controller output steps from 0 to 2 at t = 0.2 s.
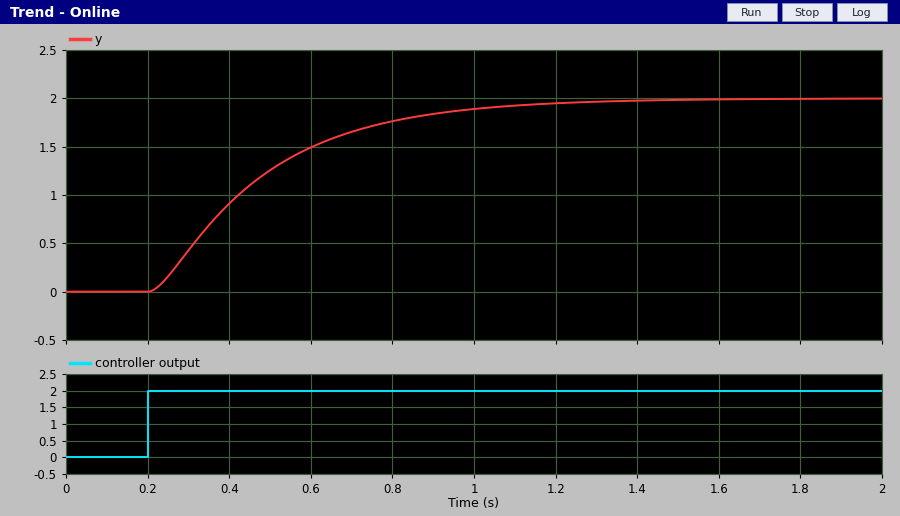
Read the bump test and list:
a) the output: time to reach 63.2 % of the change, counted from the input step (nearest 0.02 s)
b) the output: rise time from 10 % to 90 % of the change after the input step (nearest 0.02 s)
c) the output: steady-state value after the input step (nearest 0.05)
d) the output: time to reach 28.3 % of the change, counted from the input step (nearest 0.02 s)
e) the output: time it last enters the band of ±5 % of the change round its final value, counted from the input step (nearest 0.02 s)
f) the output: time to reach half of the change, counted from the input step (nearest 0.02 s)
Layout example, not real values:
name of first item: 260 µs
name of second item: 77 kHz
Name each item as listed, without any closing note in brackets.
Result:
the output: time to reach 63.2 % of the change, counted from the input step: 0.30 s
the output: rise time from 10 % to 90 % of the change after the input step: 0.58 s
the output: steady-state value after the input step: 2.00
the output: time to reach 28.3 % of the change, counted from the input step: 0.12 s
the output: time it last enters the band of ±5 % of the change round its final value, counted from the input step: 0.82 s
the output: time to reach half of the change, counted from the input step: 0.22 s
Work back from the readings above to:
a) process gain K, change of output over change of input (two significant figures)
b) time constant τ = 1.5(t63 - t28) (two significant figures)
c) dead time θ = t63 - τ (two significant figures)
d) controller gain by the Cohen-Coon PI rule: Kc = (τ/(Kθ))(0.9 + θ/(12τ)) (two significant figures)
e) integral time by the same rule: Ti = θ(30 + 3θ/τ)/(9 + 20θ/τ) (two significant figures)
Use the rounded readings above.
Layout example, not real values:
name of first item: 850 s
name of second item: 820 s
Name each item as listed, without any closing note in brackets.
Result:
process gain K, change of output over change of input: 1.0
time constant τ = 1.5(t63 - t28): 0.27 s
dead time θ = t63 - τ: 0.030 s
controller gain by the Cohen-Coon PI rule: Kc = (τ/(Kθ))(0.9 + θ/(12τ)): 8.2
integral time by the same rule: Ti = θ(30 + 3θ/τ)/(9 + 20θ/τ): 0.081 s
